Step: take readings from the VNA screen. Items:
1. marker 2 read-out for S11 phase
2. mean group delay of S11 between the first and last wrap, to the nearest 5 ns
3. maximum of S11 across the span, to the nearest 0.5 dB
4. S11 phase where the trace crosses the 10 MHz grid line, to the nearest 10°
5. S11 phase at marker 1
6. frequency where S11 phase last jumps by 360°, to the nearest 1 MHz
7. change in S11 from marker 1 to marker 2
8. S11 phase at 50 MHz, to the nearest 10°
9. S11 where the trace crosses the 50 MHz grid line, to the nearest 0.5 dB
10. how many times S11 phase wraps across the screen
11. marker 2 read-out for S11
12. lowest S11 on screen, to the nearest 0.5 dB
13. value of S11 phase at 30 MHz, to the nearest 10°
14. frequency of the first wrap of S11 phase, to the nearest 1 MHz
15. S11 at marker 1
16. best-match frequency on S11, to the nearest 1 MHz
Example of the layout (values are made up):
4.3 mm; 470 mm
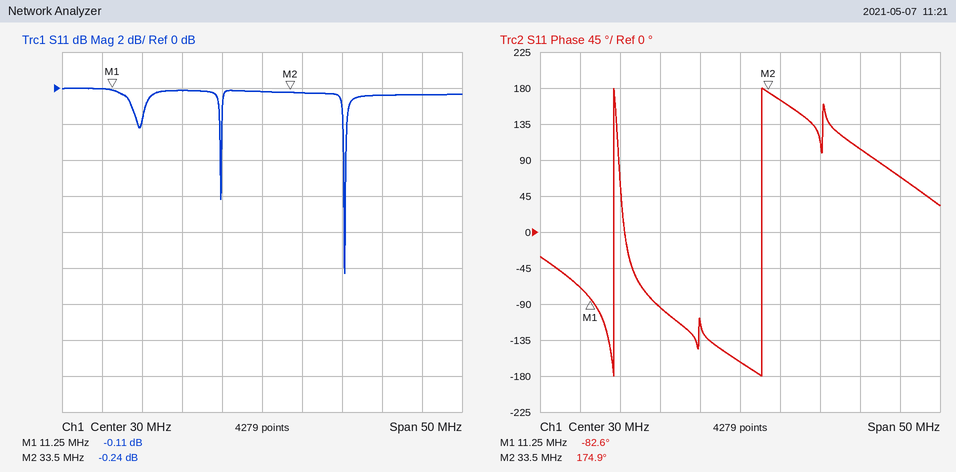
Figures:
174.9°; 55 ns; 0.0 dB; -70°; -82.6°; 33 MHz; -0.13 dB; 70°; -0.5 dB; 2; -0.24 dB; -10.5 dB; -160°; 14 MHz; -0.11 dB; 40 MHz
